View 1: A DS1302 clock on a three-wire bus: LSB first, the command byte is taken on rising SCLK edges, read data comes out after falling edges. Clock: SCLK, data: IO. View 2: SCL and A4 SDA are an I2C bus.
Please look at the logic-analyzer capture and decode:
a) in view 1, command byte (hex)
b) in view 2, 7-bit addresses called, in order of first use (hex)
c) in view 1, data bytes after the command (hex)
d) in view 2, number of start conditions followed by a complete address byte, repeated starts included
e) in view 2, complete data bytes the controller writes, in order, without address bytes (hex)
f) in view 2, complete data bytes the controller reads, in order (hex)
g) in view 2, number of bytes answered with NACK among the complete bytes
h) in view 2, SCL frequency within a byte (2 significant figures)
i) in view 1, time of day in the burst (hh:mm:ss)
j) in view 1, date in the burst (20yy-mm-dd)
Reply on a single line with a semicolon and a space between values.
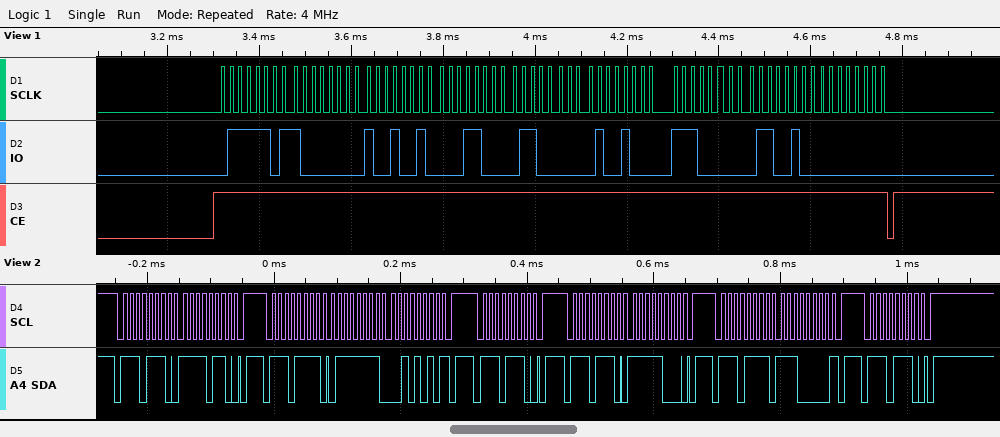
0xBE; 0x77; 01 49 18 06 12 07 26 00; 6; F6 F8; 7F 2A E0; 2; 100 kHz; 18:49:01; 2026-12-06
